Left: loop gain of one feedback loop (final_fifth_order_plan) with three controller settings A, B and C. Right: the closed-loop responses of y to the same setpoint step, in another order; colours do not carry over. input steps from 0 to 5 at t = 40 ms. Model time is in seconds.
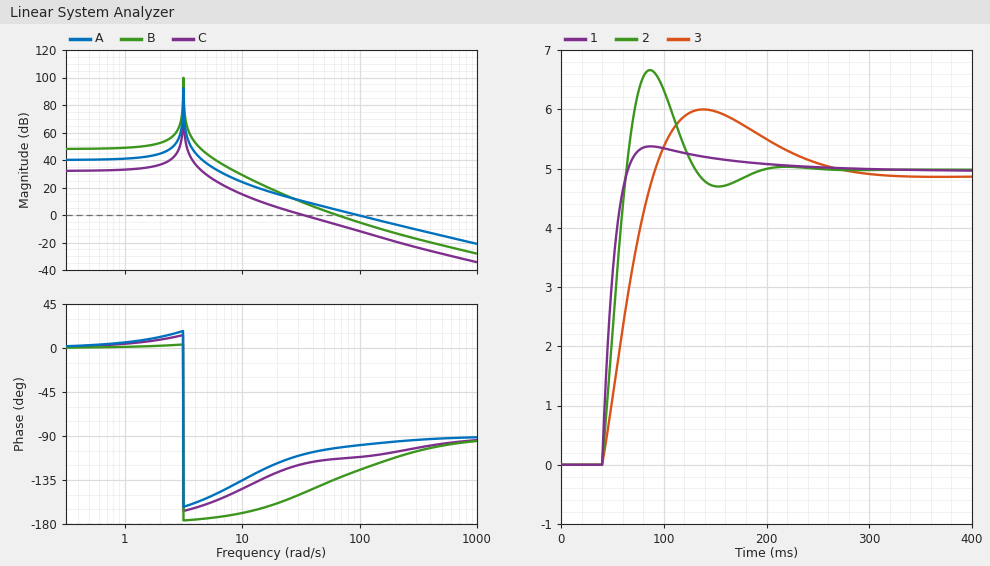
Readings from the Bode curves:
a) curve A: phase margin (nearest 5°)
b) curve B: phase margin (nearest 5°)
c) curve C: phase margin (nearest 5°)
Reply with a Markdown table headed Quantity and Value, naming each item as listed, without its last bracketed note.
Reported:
| Quantity | Value |
|---|---|
| curve A: phase margin | 80° |
| curve B: phase margin | 45° |
| curve C: phase margin | 60° |
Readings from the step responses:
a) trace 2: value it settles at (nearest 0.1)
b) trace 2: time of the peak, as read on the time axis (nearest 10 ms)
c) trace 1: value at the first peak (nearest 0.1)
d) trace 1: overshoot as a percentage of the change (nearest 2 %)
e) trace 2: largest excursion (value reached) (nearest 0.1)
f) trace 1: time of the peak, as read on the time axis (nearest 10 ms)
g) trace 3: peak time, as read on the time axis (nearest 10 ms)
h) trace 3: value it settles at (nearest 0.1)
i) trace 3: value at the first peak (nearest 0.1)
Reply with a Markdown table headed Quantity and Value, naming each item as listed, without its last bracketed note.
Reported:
| Quantity | Value |
|---|---|
| trace 2: value it settles at | 5.0 |
| trace 2: time of the peak, as read on the time axis | 90 ms |
| trace 1: value at the first peak | 5.4 |
| trace 1: overshoot as a percentage of the change | 8 % |
| trace 2: largest excursion (value reached) | 6.7 |
| trace 1: time of the peak, as read on the time axis | 90 ms |
| trace 3: peak time, as read on the time axis | 140 ms |
| trace 3: value it settles at | 4.9 |
| trace 3: value at the first peak | 6.0 |
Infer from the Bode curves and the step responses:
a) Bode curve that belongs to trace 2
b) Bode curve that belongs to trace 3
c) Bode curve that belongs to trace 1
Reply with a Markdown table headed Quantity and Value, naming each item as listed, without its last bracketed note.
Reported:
| Quantity | Value |
|---|---|
| Bode curve that belongs to trace 2 | B |
| Bode curve that belongs to trace 3 | C |
| Bode curve that belongs to trace 1 | A |
